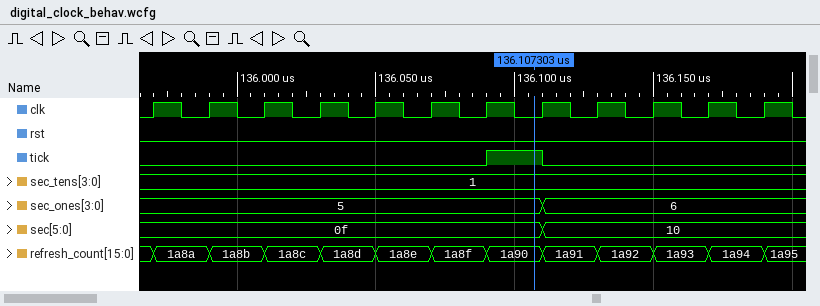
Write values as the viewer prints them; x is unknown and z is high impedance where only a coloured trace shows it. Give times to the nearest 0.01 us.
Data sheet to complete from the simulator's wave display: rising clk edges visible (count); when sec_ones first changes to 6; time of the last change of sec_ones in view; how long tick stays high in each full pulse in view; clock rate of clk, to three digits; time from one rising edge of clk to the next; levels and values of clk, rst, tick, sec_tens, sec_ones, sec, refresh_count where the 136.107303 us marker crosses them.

12
136.11 us
136.11 us
0.02 us
50.0 MHz
0.02 us
clk=0, rst=0, tick=1, sec_tens=1, sec_ones=5, sec=0f, refresh_count=1a90
